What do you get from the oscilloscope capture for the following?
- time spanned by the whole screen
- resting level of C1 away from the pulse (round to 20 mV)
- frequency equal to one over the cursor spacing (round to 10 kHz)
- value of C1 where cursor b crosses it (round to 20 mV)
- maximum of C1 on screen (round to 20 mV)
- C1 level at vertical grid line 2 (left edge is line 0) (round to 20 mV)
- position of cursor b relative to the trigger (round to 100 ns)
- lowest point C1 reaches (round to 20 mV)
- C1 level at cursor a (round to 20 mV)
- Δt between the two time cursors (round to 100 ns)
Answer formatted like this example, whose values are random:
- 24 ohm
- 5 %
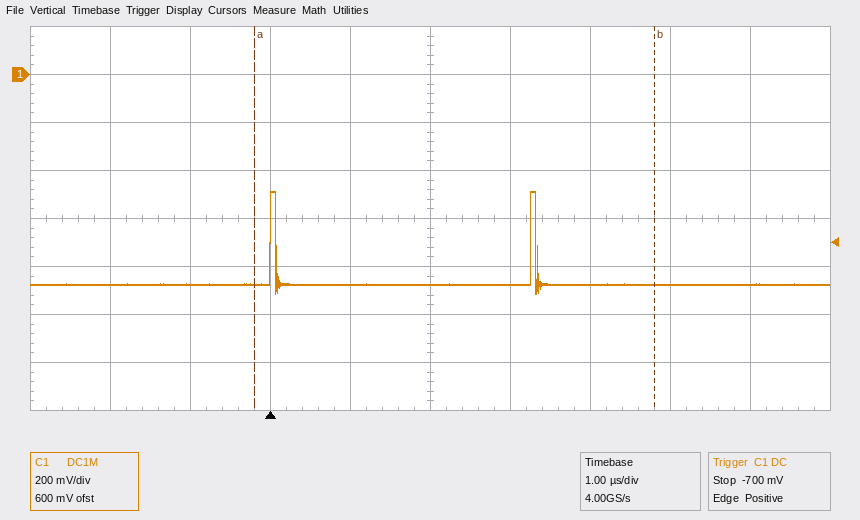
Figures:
- 10 µs
- -880 mV
- 200 kHz
- -880 mV
- -480 mV
- -880 mV
- +4.8 µs
- -920 mV
- -880 mV
- 5.0 µs
